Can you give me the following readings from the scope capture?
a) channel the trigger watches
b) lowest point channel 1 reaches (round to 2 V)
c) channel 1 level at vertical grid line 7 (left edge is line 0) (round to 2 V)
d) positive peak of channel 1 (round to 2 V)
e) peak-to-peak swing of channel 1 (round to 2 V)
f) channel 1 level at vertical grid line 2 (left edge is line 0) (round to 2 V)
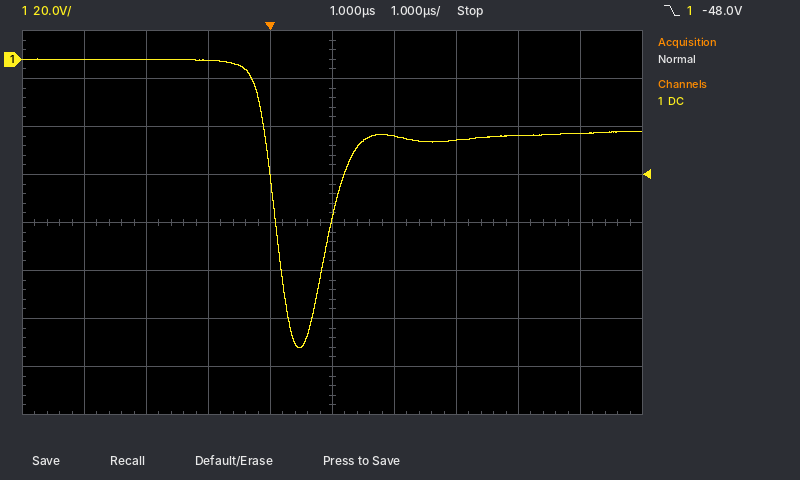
channel 1
-120 V
-34 V
0 V
120 V
0 V
